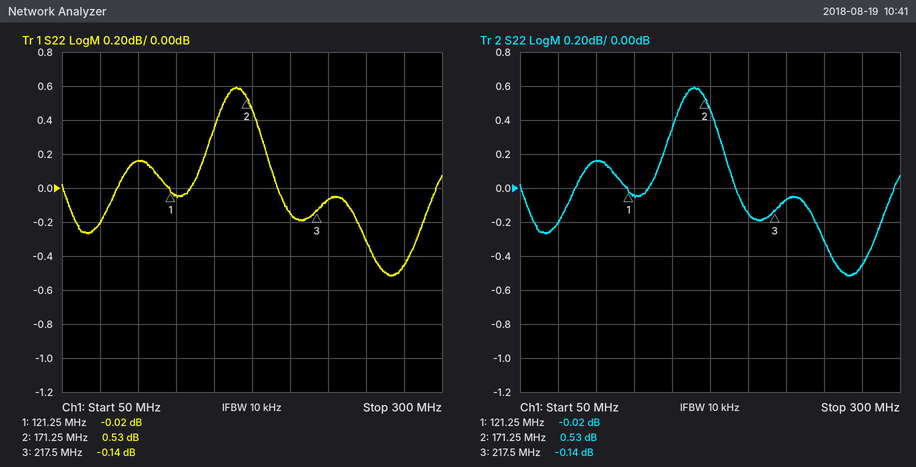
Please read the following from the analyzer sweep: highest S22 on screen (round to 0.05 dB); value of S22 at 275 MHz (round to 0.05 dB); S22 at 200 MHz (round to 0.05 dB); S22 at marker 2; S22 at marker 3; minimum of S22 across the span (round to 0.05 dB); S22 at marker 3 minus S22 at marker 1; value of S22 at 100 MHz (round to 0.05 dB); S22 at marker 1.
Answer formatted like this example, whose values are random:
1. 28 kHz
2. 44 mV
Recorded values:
1. 0.60 dB
2. -0.45 dB
3. -0.15 dB
4. 0.53 dB
5. -0.14 dB
6. -0.50 dB
7. -0.12 dB
8. 0.15 dB
9. -0.02 dB
